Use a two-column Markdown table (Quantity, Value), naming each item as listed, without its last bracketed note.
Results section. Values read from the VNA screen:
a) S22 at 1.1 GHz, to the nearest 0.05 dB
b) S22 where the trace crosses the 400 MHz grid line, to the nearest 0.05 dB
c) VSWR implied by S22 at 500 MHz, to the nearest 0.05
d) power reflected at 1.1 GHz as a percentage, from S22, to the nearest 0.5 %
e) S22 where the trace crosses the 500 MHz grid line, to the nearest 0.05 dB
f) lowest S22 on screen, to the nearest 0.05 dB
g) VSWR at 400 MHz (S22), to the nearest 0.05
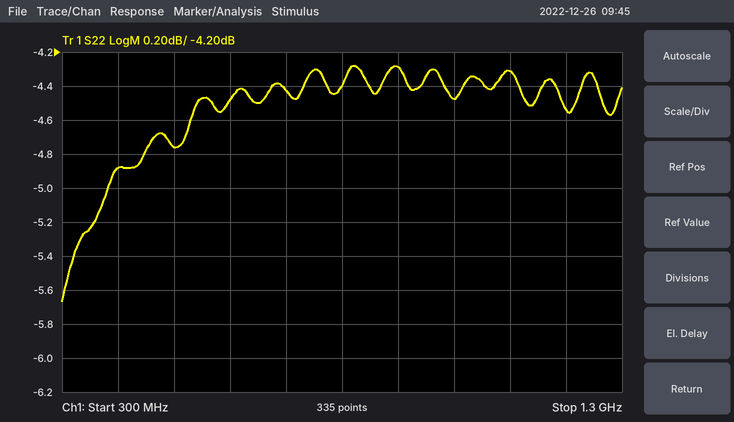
| Quantity | Value |
|---|---|
| S22 at 1.1 GHz, to the nearest 0.05 dB | -4.30 dB |
| S22 where the trace crosses the 400 MHz grid line, to the nearest 0.05 dB | -4.90 dB |
| VSWR implied by S22 at 500 MHz, to the nearest 0.05 | 3.75 |
| power reflected at 1.1 GHz as a percentage, from S22, to the nearest 0.5 % | 37.0 % |
| S22 where the trace crosses the 500 MHz grid line, to the nearest 0.05 dB | -4.75 dB |
| lowest S22 on screen, to the nearest 0.05 dB | -5.65 dB |
| VSWR at 400 MHz (S22), to the nearest 0.05 | 3.65 |
